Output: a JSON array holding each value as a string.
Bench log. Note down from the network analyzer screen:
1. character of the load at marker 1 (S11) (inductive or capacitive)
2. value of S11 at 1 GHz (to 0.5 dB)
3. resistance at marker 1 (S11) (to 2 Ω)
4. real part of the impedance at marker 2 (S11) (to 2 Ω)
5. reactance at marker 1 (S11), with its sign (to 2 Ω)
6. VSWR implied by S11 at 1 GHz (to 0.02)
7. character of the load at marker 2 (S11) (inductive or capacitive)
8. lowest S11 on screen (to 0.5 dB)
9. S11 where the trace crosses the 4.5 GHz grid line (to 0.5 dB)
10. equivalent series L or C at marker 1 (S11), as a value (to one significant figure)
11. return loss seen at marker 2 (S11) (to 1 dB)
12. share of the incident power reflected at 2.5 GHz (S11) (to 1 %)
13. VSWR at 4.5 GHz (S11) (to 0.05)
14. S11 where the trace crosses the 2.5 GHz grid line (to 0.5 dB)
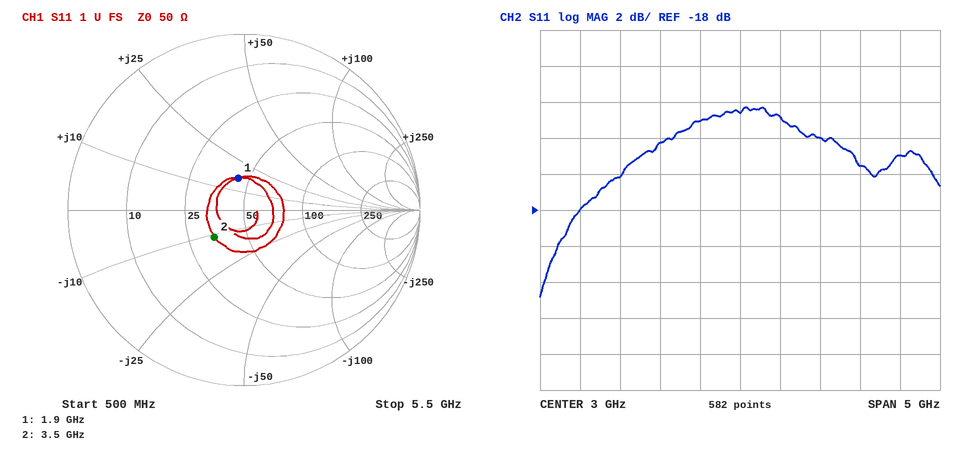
["inductive", "-18.0 dB", "44 Ω", "34 Ω", "+16 Ω", "1.28", "capacitive", "-23.0 dB", "-15.5 dB", "1 nH", "13 dB", "5 %", "1.40", "-13.0 dB"]
